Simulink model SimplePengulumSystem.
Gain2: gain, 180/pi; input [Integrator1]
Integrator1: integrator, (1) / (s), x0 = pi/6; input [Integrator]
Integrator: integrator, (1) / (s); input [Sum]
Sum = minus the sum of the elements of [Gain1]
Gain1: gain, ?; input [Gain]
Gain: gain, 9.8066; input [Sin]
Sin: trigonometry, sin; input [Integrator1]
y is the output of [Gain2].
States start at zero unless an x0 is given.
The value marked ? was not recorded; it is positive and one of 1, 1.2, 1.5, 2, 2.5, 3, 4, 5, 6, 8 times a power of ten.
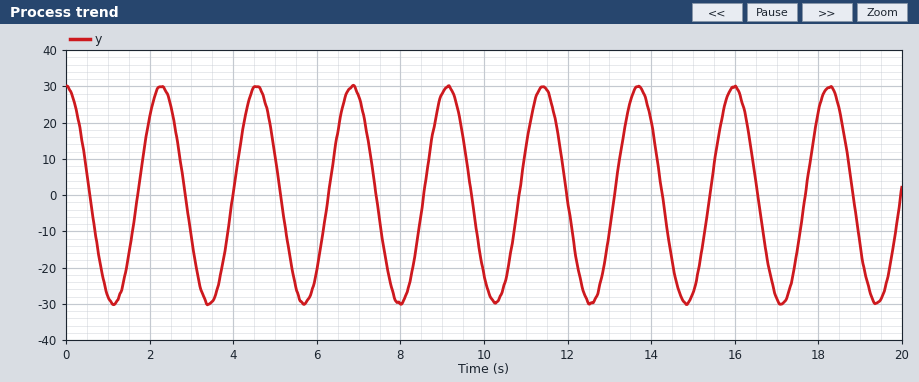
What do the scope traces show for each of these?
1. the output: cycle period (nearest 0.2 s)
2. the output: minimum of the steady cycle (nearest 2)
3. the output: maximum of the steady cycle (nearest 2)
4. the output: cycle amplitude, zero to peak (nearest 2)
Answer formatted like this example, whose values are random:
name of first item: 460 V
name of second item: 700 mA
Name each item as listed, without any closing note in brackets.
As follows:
the output: cycle period: 2.2 s
the output: minimum of the steady cycle: -30
the output: maximum of the steady cycle: 30
the output: cycle amplitude, zero to peak: 30
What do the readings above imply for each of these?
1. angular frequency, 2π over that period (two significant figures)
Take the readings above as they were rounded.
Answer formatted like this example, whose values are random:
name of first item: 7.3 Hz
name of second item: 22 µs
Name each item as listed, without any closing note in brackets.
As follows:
angular frequency, 2π over that period: 2.9 rad/s
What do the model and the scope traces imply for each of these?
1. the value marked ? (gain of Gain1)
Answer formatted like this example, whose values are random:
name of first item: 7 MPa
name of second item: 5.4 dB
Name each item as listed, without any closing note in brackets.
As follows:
the value marked ?: 0.8
